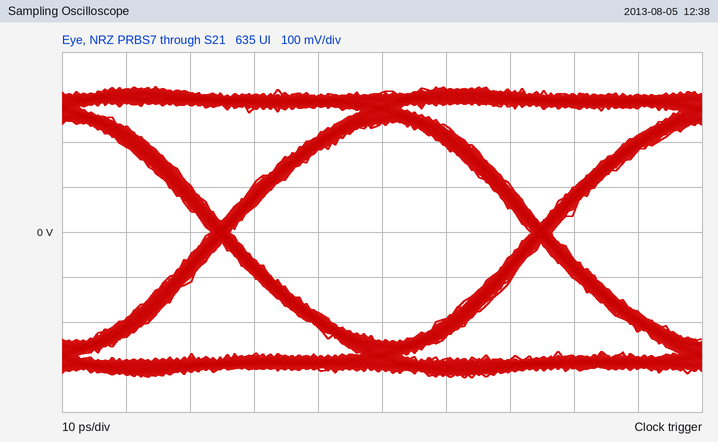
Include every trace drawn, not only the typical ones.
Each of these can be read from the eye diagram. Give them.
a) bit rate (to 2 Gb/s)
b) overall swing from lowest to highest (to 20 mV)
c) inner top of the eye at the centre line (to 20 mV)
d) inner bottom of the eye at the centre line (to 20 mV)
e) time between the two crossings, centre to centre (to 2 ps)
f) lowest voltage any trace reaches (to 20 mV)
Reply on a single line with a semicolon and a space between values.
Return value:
20 Gb/s; 640 mV; 240 mV; -240 mV; 50 ps; -320 mV
